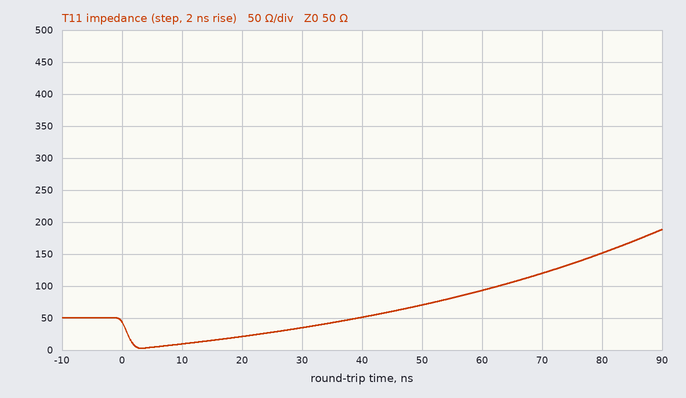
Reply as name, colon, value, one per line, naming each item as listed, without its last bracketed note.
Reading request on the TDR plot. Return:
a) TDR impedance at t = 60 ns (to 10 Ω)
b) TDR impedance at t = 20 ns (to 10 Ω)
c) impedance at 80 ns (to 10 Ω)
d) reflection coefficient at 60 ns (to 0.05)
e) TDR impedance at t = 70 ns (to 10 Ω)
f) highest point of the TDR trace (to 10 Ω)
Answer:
TDR impedance at t = 60 ns: 90 Ω
TDR impedance at t = 20 ns: 20 Ω
impedance at 80 ns: 150 Ω
reflection coefficient at 60 ns: +0.30
TDR impedance at t = 70 ns: 120 Ω
highest point of the TDR trace: 190 Ω
